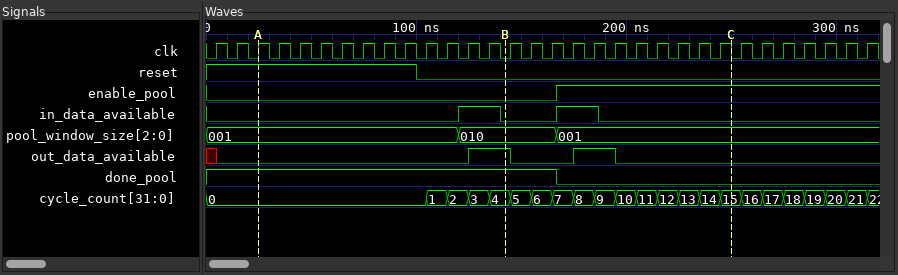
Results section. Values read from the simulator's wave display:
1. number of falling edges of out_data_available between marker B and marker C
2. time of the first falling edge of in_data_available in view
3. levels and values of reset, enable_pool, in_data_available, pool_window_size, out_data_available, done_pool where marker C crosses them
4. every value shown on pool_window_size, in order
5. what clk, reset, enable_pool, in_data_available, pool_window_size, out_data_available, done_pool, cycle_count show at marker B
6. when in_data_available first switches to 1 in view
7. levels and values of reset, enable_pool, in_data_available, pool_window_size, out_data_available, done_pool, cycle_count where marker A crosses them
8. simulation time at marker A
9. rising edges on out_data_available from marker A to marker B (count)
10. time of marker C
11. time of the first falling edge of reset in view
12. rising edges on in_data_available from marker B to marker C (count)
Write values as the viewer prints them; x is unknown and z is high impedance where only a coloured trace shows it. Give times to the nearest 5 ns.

2
140 ns
reset=0, enable_pool=1, in_data_available=0, pool_window_size=001, out_data_available=0, done_pool=0
001, 010, 001
clk=0, reset=0, enable_pool=0, in_data_available=0, pool_window_size=010, out_data_available=1, done_pool=1, cycle_count=4
120 ns
reset=1, enable_pool=0, in_data_available=0, pool_window_size=001, out_data_available=0, done_pool=1, cycle_count=0
25 ns
1
250 ns
100 ns
1
